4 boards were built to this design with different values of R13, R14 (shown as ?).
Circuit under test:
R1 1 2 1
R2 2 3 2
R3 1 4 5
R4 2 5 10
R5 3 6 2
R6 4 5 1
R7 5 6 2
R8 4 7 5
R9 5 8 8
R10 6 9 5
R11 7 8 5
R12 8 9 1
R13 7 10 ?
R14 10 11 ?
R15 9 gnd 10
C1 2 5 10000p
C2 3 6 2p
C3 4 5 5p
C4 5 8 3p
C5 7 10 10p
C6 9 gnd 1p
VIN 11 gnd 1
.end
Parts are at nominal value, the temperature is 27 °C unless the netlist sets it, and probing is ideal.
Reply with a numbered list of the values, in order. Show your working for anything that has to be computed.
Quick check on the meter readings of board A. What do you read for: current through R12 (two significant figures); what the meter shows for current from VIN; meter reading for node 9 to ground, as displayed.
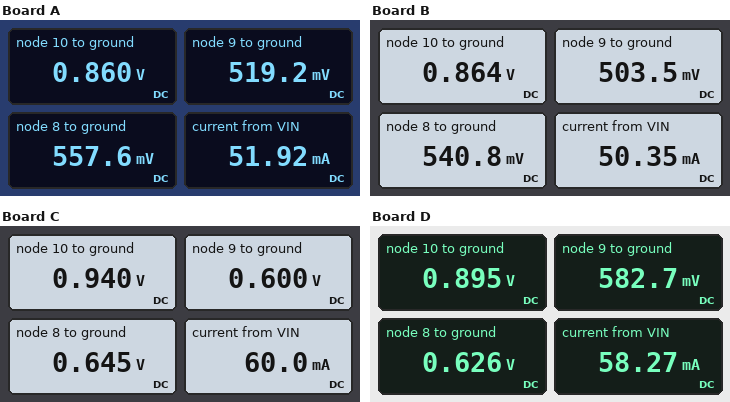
1. (557.6 mV - 519.2 mV) / 1 Ω = 38 mA
2. 51.92 mA
3. 519.2 mV
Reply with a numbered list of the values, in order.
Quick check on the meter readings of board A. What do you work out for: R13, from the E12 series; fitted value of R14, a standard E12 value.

1. 2.7 Ω
2. 2.7 Ω
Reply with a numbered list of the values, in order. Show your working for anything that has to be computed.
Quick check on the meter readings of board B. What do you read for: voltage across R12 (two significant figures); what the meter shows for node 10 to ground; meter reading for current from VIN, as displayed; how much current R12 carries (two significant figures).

1. 540.8 mV - 503.5 mV = 37 mV
2. 0.864 V
3. 50.35 mA
4. (540.8 mV - 503.5 mV) / 1 Ω = 37 mA
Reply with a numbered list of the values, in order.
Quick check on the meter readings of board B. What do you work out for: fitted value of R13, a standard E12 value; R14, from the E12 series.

1. 3.3 Ω
2. 2.7 Ω
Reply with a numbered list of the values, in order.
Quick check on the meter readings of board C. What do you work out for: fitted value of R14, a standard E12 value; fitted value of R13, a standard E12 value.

1. 1 Ω
2. 1.8 Ω
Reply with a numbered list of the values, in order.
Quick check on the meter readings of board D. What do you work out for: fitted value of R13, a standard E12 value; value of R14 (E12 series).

1. 1.5 Ω
2. 1.8 Ω
